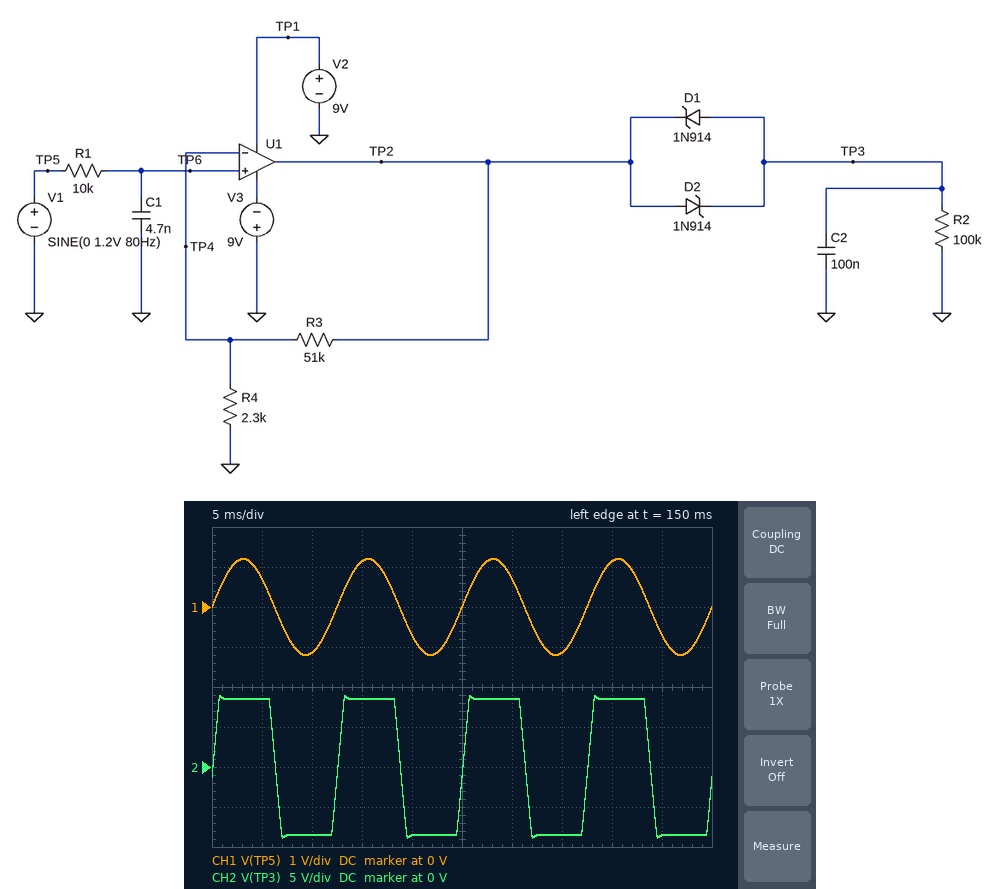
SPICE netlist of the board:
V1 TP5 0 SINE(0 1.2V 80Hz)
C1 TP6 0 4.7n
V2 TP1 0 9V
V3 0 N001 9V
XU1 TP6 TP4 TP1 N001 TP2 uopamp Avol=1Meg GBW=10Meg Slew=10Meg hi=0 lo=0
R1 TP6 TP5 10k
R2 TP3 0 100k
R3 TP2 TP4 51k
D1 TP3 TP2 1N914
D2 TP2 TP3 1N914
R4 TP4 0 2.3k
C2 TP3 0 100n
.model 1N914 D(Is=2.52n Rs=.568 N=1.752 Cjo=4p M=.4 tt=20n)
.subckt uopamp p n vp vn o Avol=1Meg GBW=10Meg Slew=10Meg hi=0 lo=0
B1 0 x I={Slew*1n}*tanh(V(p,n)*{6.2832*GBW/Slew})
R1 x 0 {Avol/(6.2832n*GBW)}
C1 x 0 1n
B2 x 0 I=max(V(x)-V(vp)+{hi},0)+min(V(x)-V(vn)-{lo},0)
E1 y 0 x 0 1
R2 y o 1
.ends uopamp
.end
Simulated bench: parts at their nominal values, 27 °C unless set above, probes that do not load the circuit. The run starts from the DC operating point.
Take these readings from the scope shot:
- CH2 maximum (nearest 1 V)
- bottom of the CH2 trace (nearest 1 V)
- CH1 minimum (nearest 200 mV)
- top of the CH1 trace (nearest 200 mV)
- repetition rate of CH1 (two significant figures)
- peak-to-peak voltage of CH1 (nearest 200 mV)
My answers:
9 V
-9 V
-1.2 V
1.2 V
80 Hz
2.4 V
